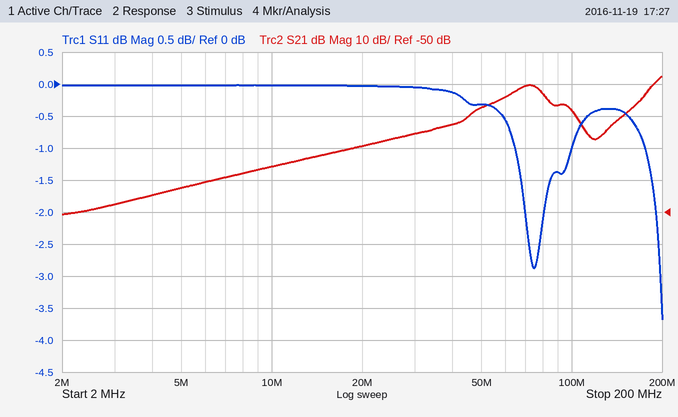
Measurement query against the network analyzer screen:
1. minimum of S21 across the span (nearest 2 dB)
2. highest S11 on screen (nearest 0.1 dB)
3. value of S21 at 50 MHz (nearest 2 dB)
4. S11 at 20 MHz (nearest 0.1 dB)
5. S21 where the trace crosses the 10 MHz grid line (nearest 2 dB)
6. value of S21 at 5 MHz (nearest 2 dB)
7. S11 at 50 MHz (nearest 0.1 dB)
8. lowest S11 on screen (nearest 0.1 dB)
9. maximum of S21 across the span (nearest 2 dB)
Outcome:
-50 dB
0.0 dB
-18 dB
0.0 dB
-36 dB
-42 dB
-0.3 dB
-3.7 dB
-8 dB
